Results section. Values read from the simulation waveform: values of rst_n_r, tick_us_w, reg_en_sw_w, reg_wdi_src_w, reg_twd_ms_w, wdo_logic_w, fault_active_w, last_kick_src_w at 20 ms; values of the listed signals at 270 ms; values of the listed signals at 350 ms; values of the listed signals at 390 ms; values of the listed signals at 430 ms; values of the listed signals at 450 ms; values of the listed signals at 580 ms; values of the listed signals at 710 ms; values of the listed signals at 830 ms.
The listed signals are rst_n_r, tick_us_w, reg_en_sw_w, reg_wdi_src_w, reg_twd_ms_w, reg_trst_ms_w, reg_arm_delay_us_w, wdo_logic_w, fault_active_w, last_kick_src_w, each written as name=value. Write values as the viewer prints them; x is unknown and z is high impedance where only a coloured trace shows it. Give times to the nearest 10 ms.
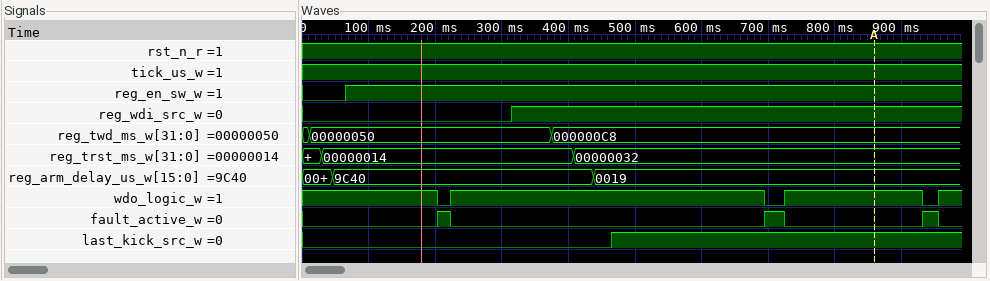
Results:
rst_n_r=1, tick_us_w=1, reg_en_sw_w=0, reg_wdi_src_w=0, reg_twd_ms_w=00000050, wdo_logic_w=1, fault_active_w=0, last_kick_src_w=0
rst_n_r=1, tick_us_w=1, reg_en_sw_w=1, reg_wdi_src_w=0, reg_twd_ms_w=00000050, reg_trst_ms_w=00000014, reg_arm_delay_us_w=9C40, wdo_logic_w=1, fault_active_w=0, last_kick_src_w=0
rst_n_r=1, tick_us_w=1, reg_en_sw_w=1, reg_wdi_src_w=1, reg_twd_ms_w=00000050, reg_trst_ms_w=00000014, reg_arm_delay_us_w=9C40, wdo_logic_w=1, fault_active_w=0, last_kick_src_w=0
rst_n_r=1, tick_us_w=1, reg_en_sw_w=1, reg_wdi_src_w=1, reg_twd_ms_w=000000C8, reg_trst_ms_w=00000014, reg_arm_delay_us_w=9C40, wdo_logic_w=1, fault_active_w=0, last_kick_src_w=0
rst_n_r=1, tick_us_w=1, reg_en_sw_w=1, reg_wdi_src_w=1, reg_twd_ms_w=000000C8, reg_trst_ms_w=00000032, reg_arm_delay_us_w=9C40, wdo_logic_w=1, fault_active_w=0, last_kick_src_w=0
rst_n_r=1, tick_us_w=1, reg_en_sw_w=1, reg_wdi_src_w=1, reg_twd_ms_w=000000C8, reg_trst_ms_w=00000032, reg_arm_delay_us_w=0019, wdo_logic_w=1, fault_active_w=0, last_kick_src_w=0
rst_n_r=1, tick_us_w=1, reg_en_sw_w=1, reg_wdi_src_w=1, reg_twd_ms_w=000000C8, reg_trst_ms_w=00000032, reg_arm_delay_us_w=0019, wdo_logic_w=1, fault_active_w=0, last_kick_src_w=1
rst_n_r=1, tick_us_w=1, reg_en_sw_w=1, reg_wdi_src_w=1, reg_twd_ms_w=000000C8, reg_trst_ms_w=00000032, reg_arm_delay_us_w=0019, wdo_logic_w=0, fault_active_w=1, last_kick_src_w=1
rst_n_r=1, tick_us_w=1, reg_en_sw_w=1, reg_wdi_src_w=1, reg_twd_ms_w=000000C8, reg_trst_ms_w=00000032, reg_arm_delay_us_w=0019, wdo_logic_w=1, fault_active_w=0, last_kick_src_w=1
